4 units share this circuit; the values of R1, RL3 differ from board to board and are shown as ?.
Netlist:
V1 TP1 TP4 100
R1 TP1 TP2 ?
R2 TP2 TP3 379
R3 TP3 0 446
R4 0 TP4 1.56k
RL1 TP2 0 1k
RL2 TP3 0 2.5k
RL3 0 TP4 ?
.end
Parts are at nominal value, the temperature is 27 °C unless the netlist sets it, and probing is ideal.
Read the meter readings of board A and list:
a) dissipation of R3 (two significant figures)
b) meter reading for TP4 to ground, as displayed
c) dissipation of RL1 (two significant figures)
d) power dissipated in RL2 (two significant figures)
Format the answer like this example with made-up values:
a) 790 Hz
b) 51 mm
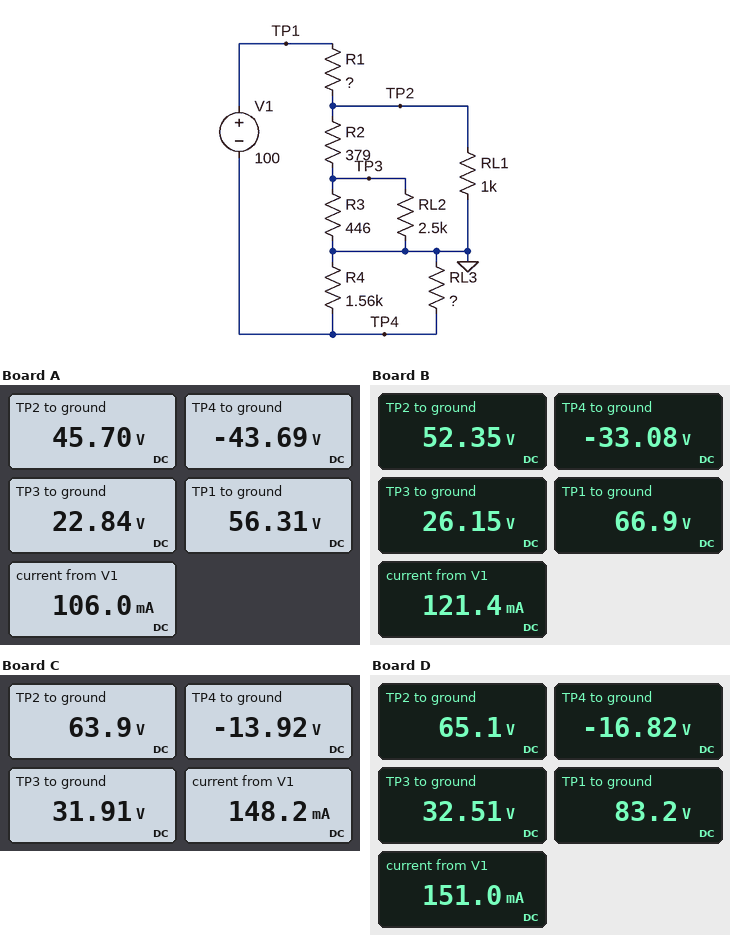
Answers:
a) 1.2 W
b) -43.69 V
c) 2.1 W
d) 210 mW
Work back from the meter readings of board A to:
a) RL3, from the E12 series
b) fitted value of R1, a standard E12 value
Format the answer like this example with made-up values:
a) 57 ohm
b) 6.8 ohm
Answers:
a) 560 Ω
b) 100 Ω
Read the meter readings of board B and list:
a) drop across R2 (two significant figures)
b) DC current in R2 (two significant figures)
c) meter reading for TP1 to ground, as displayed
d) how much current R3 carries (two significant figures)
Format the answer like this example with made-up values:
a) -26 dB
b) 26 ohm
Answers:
a) 26 V
b) 69 mA
c) 66.9 V
d) 59 mA
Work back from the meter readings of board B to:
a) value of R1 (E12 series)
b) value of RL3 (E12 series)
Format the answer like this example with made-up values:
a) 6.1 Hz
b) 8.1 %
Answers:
a) 120 Ω
b) 330 Ω
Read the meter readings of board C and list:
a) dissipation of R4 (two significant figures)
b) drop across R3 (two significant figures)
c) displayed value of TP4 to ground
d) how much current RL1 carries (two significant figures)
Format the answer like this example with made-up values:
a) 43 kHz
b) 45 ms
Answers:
a) 120 mW
b) 32 V
c) -13.92 V
d) 64 mA
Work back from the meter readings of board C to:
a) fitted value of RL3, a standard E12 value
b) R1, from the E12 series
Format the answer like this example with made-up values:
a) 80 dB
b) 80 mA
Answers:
a) 100 Ω
b) 150 Ω
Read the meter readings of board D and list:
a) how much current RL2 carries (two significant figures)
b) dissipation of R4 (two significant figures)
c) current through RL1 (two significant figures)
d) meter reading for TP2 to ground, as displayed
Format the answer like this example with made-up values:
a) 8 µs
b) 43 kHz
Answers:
a) 13 mA
b) 180 mW
c) 65 mA
d) 65.1 V
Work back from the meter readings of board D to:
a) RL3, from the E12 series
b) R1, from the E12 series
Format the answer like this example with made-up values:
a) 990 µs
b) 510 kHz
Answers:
a) 120 Ω
b) 120 Ω
